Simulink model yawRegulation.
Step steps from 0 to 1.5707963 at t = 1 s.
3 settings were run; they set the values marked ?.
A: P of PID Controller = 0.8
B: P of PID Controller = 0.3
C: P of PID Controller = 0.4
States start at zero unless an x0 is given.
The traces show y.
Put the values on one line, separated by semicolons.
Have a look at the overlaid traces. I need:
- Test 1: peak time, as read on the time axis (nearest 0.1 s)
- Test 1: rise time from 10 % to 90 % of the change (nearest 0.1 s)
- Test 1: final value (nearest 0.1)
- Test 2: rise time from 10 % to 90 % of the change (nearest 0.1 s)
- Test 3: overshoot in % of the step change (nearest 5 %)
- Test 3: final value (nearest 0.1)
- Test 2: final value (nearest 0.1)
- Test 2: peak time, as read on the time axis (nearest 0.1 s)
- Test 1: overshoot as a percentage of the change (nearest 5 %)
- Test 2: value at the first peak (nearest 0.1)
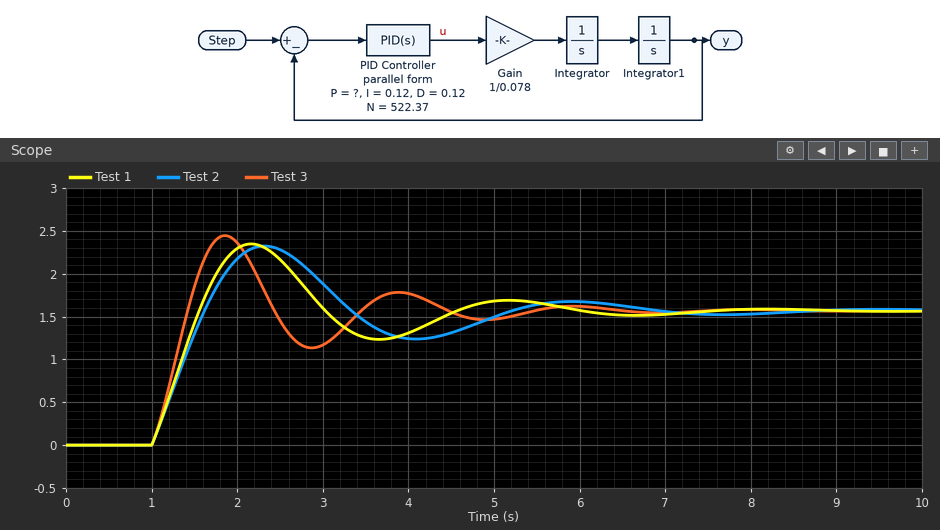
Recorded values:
2.2 s; 0.4 s; 1.6; 0.5 s; 55 %; 1.6; 1.6; 2.3 s; 50 %; 2.3
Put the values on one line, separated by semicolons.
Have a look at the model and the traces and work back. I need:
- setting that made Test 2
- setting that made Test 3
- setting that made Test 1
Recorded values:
B; A; C
